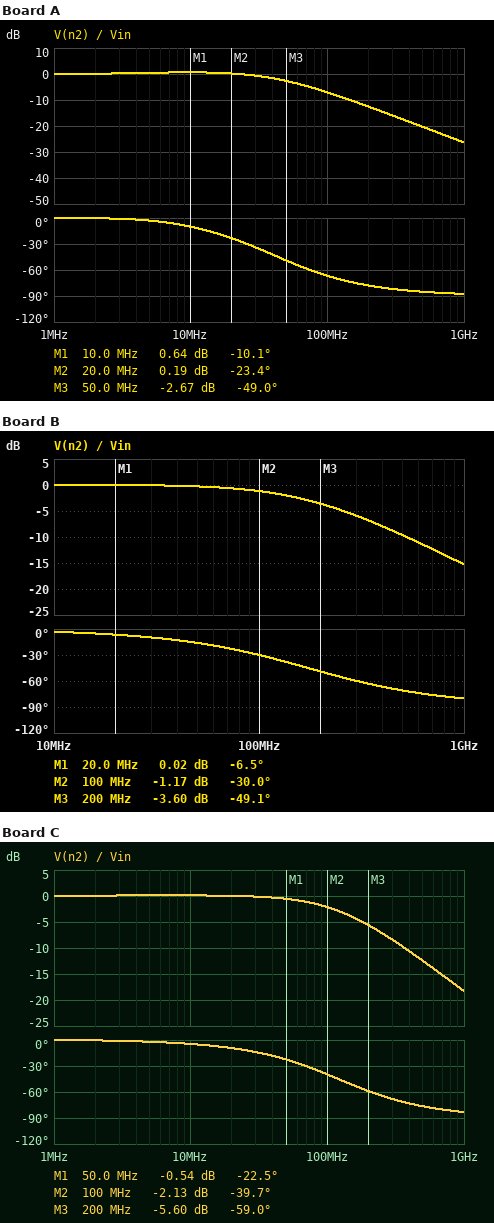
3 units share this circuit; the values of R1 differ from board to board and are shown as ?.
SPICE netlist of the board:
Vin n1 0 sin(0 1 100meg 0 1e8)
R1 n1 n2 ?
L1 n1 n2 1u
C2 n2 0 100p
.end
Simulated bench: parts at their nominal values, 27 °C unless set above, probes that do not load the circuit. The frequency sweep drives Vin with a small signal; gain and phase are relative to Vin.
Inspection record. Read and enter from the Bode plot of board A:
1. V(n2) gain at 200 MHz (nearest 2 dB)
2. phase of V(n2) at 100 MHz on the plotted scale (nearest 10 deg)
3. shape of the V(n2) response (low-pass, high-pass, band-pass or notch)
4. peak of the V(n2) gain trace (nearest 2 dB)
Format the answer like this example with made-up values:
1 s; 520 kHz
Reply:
-12 dB; -70 deg; low-pass; 0 dB
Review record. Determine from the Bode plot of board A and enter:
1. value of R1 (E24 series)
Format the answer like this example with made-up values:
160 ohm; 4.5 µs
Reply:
33 Ω
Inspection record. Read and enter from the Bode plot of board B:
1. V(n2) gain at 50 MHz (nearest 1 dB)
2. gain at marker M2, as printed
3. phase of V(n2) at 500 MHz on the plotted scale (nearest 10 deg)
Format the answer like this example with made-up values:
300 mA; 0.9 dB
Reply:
0 dB; -1.17 dB; -70 deg
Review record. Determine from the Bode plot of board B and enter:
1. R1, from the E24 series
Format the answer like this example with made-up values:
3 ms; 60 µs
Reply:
9.1 Ω
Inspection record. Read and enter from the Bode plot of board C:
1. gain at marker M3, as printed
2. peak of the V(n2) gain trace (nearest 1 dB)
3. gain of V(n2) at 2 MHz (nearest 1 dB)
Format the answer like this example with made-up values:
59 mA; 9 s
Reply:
-5.60 dB; 0 dB; 0 dB
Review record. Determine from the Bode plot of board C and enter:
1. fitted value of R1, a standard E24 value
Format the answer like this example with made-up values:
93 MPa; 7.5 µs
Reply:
13 Ω
